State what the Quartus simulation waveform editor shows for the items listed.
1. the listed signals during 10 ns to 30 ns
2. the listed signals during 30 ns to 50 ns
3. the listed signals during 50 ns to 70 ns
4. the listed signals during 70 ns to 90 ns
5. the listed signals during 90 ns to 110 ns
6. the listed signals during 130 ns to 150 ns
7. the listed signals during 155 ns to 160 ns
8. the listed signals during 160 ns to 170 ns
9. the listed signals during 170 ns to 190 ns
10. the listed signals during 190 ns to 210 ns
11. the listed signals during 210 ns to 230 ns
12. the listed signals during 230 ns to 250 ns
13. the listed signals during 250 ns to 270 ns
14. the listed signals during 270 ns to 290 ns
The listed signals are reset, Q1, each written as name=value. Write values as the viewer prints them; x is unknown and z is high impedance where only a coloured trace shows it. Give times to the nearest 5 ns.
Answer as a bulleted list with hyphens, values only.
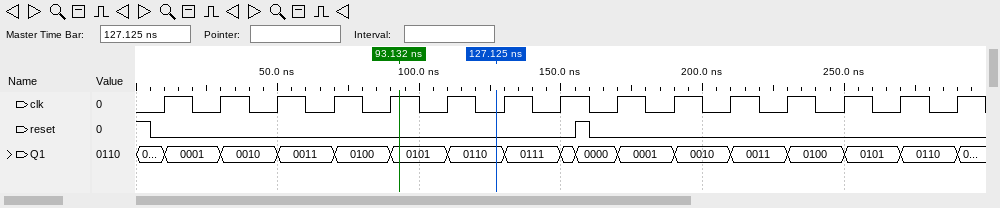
- reset=0, Q1=0001
- reset=0, Q1=0010
- reset=0, Q1=0011
- reset=0, Q1=0100
- reset=0, Q1=0101
- reset=0, Q1=0111
- reset=1, Q1=0000
- reset=0, Q1=0000
- reset=0, Q1=0001
- reset=0, Q1=0010
- reset=0, Q1=0011
- reset=0, Q1=0100
- reset=0, Q1=0101
- reset=0, Q1=0110
